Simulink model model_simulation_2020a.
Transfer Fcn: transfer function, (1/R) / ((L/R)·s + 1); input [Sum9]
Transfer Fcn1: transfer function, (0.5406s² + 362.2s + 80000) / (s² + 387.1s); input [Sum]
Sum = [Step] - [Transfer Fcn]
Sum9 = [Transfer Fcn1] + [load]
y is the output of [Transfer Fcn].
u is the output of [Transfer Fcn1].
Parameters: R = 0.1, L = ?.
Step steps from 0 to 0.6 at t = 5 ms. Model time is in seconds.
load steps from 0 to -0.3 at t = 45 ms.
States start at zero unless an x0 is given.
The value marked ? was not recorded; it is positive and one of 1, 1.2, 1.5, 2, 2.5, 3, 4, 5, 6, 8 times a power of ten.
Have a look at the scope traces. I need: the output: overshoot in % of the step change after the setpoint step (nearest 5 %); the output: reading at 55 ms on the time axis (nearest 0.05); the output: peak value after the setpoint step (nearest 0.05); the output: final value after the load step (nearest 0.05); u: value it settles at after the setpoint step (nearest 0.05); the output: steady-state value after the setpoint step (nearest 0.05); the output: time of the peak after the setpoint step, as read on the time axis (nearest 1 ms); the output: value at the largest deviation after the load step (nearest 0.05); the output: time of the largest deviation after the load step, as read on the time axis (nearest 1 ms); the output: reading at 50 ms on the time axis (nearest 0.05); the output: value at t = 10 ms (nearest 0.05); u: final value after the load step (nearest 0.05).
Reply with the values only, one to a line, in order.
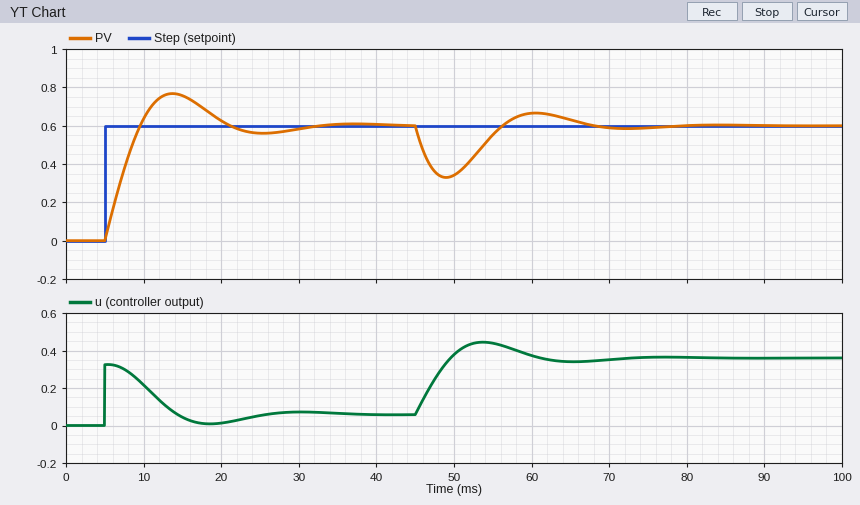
30 %
0.55
0.75
0.60
0.05
0.60
14 ms
0.35
49 ms
0.35
0.65
0.35
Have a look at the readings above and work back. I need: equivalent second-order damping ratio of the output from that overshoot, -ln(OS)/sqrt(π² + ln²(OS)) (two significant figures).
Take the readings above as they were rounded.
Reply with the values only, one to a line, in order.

0.36
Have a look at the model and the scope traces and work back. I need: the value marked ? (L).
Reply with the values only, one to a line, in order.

0.002
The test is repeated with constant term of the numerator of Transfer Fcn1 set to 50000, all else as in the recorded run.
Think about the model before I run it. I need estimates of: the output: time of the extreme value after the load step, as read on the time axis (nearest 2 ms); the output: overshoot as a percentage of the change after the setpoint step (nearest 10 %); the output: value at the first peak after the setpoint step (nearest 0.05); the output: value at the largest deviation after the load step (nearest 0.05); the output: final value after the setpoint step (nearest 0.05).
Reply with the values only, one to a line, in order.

50 ms
20 %
0.70
0.30
0.60
